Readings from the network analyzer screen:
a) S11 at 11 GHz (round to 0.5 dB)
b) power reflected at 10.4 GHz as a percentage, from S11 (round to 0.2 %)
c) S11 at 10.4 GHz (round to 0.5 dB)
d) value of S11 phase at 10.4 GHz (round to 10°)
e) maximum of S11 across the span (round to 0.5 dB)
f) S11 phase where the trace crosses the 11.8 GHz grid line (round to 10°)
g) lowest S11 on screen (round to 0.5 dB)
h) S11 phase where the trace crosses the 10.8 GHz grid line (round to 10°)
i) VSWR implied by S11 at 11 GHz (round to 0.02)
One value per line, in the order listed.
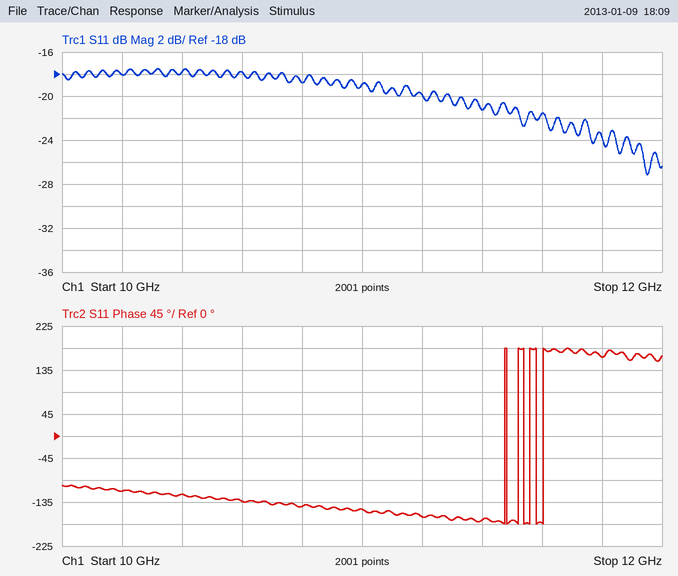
-19.0 dB
1.6 %
-18.0 dB
-120°
-17.5 dB
160°
-27.0 dB
-140°
1.26
